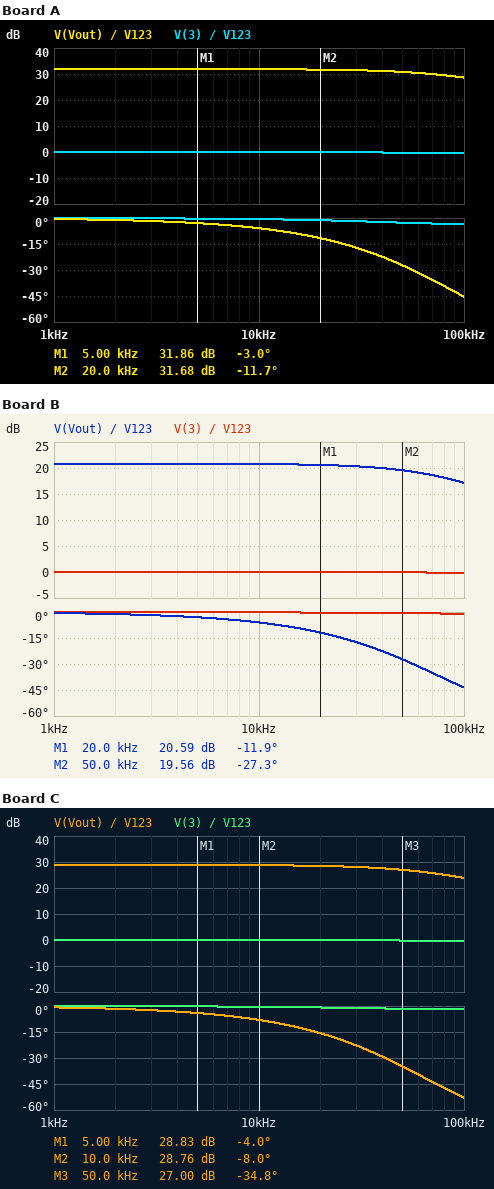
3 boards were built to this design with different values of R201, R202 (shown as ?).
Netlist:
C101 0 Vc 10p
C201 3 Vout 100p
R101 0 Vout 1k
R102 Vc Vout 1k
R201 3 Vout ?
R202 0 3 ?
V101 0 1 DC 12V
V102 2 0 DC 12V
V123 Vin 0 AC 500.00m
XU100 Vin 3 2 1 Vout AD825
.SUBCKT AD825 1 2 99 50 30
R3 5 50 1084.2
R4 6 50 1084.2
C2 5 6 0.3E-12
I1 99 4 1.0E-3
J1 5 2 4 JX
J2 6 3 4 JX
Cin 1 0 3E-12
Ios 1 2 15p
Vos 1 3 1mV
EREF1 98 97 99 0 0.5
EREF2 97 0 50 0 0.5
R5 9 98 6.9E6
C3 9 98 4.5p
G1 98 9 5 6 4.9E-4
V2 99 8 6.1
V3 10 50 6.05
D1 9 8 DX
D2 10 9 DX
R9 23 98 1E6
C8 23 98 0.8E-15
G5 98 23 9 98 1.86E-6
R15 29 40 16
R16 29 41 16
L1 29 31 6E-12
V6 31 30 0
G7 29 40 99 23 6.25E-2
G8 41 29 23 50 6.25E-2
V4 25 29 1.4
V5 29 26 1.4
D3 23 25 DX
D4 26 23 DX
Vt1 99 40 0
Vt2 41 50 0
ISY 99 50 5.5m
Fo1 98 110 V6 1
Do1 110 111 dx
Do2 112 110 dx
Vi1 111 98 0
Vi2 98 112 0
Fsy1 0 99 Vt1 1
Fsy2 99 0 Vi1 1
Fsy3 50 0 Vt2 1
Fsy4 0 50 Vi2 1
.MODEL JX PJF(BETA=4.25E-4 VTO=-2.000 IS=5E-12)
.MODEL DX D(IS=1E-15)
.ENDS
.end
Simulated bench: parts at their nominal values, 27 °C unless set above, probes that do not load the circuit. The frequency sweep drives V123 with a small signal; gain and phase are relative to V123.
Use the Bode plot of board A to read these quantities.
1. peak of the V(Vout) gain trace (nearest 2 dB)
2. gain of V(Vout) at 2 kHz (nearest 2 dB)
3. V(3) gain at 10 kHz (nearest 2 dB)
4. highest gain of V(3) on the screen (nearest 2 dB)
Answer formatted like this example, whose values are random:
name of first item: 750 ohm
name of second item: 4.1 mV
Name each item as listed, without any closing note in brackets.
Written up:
peak of the V(Vout) gain trace: 32 dB
gain of V(Vout) at 2 kHz: 32 dB
V(3) gain at 10 kHz: 0 dB
highest gain of V(3) on the screen: 0 dB
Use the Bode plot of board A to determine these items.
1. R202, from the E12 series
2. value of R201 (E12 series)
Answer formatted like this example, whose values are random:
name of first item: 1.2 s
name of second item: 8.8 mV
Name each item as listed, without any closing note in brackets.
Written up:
R202, from the E12 series: 390 Ω
value of R201: 15 kΩ
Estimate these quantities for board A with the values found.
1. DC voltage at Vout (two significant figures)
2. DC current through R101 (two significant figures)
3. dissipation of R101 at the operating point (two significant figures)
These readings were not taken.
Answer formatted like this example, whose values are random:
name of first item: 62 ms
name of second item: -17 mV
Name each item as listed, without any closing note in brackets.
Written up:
DC voltage at Vout: -39 mV
DC current through R101: 39 µA
dissipation of R101 at the operating point: 1.5 µW
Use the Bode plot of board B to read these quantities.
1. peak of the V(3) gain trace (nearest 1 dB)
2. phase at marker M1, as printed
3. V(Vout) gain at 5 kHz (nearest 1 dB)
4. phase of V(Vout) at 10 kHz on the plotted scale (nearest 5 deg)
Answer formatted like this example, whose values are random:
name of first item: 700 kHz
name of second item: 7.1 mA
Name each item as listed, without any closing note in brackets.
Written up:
peak of the V(3) gain trace: 0 dB
phase at marker M1, as printed: -11.9 deg
V(Vout) gain at 5 kHz: 21 dB
phase of V(Vout) at 10 kHz on the plotted scale: -5 deg
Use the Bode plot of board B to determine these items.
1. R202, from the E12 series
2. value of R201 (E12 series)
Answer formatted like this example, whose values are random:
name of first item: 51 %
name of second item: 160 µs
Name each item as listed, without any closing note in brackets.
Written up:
R202, from the E12 series: 1.8 kΩ
value of R201: 18 kΩ
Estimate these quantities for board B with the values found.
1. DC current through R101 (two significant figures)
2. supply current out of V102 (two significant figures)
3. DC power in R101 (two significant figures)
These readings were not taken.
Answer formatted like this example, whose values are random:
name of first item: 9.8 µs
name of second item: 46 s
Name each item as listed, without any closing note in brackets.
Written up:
DC current through R101: 11 µA
supply current out of V102: 6.5 mA
DC power in R101: 120 nW
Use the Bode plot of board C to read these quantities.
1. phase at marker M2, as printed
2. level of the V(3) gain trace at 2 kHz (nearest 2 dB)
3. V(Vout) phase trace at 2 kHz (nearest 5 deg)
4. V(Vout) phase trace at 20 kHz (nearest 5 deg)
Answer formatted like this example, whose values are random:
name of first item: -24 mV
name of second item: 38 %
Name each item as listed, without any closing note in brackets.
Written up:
phase at marker M2, as printed: -8.0 deg
level of the V(3) gain trace at 2 kHz: 0 dB
V(Vout) phase trace at 2 kHz: 0 deg
V(Vout) phase trace at 20 kHz: -15 deg
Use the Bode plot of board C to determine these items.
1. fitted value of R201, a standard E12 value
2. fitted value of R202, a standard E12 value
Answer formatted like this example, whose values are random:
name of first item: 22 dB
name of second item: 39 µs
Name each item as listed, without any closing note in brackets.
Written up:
fitted value of R201, a standard E12 value: 22 kΩ
fitted value of R202, a standard E12 value: 820 Ω
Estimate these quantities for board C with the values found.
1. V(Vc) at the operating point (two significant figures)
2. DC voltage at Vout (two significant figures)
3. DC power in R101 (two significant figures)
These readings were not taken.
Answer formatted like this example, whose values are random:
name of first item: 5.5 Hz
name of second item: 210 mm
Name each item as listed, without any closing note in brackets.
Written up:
V(Vc) at the operating point: -28 mV
DC voltage at Vout: -28 mV
DC power in R101: 770 nW
